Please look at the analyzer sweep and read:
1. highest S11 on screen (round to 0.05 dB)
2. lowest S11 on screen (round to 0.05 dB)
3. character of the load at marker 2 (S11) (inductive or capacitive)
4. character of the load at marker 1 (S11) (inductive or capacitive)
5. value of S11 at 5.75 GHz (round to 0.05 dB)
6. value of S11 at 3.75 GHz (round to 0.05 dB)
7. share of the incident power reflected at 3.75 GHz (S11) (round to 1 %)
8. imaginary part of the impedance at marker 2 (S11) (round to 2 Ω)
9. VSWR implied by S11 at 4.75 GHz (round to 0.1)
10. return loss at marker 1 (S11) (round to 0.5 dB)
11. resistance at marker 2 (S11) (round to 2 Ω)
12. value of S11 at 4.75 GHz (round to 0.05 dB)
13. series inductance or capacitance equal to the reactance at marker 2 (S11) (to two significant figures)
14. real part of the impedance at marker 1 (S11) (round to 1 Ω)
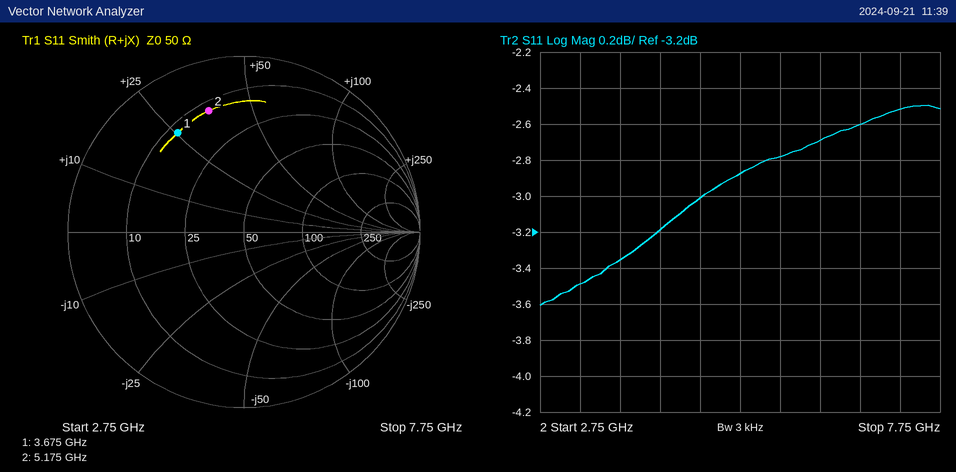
-2.50 dB
-3.60 dB
inductive
inductive
-2.80 dB
-3.35 dB
46 %
+36 Ω
5.8
3.5 dB
12 Ω
-3.00 dB
1.1 nH
12 Ω
